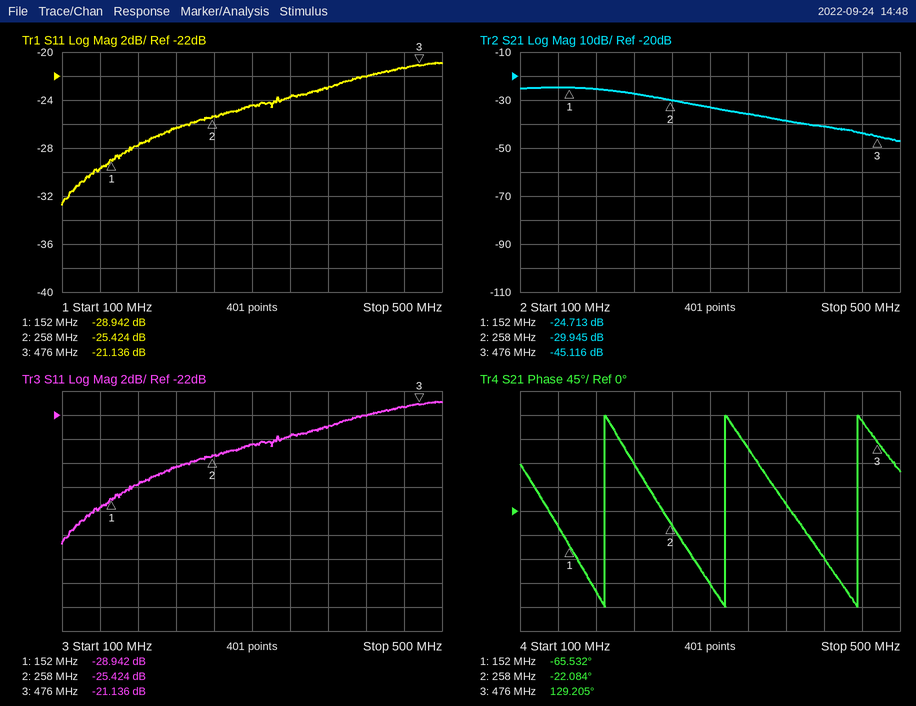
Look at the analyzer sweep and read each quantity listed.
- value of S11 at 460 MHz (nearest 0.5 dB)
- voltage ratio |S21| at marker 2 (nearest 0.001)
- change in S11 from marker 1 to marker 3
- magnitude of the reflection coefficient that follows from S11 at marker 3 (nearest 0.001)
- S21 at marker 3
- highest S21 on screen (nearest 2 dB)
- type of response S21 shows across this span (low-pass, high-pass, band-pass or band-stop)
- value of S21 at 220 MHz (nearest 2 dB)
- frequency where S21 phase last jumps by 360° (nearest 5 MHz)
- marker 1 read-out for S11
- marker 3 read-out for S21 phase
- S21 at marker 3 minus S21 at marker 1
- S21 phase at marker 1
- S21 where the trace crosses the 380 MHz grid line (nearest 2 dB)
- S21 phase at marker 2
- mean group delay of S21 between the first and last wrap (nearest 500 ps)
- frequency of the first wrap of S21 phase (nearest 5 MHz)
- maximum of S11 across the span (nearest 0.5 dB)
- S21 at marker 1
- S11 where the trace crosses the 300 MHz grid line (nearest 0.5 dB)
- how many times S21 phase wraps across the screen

-21.5 dB
0.032
7.806 dB
0.088
-45.116 dB
-24 dB
low-pass
-28 dB
455 MHz
-28.942 dB
129.205°
-20.403 dB
-65.532°
-38 dB
-22.084°
7.5 ns
190 MHz
-21.0 dB
-24.713 dB
-24.5 dB
3
